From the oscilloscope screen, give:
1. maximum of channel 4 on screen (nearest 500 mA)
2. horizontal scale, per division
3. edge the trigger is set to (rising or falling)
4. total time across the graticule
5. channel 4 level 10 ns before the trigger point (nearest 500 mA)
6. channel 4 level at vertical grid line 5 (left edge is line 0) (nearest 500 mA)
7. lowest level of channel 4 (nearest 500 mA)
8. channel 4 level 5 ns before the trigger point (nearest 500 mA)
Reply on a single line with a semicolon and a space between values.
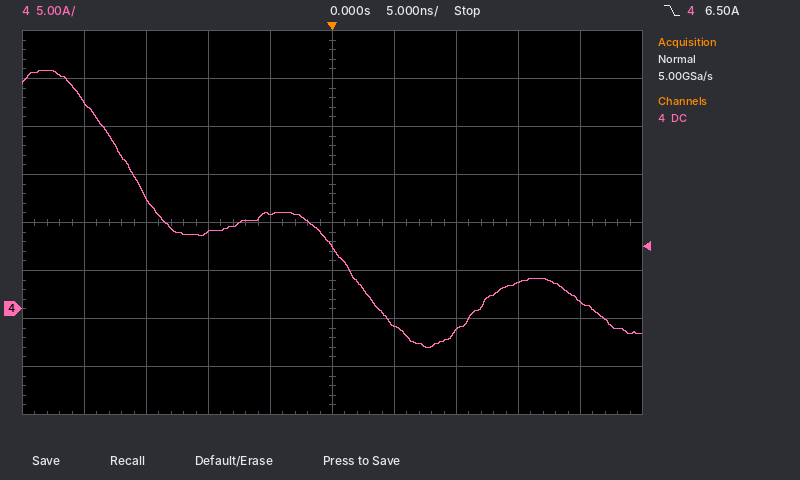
25.0 A; 5 ns; falling; 50 ns; 8.0 A; 6.5 A; -4.0 A; 10.0 A
